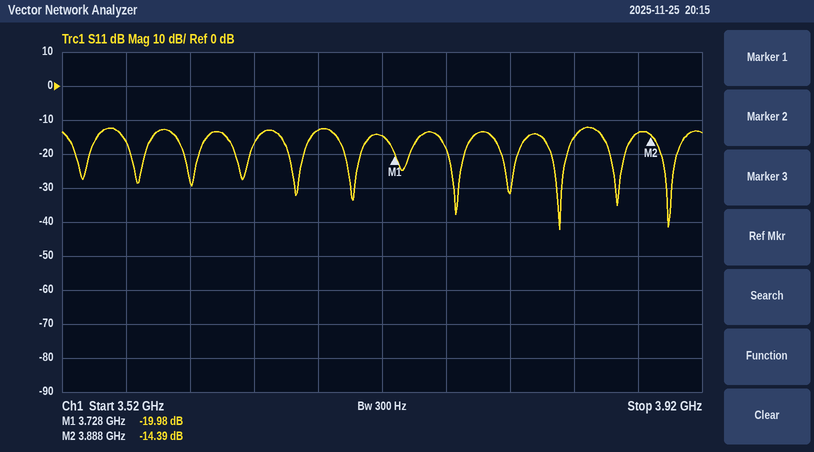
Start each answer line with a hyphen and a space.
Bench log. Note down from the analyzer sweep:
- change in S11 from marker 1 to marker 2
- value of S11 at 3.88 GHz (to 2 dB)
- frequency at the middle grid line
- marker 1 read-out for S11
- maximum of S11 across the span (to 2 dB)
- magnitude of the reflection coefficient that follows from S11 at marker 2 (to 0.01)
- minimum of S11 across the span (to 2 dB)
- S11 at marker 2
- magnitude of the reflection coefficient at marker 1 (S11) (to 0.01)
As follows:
- 5.59 dB
- -14 dB
- 3.72 GHz
- -19.98 dB
- -12 dB
- 0.19
- -42 dB
- -14.39 dB
- 0.10
